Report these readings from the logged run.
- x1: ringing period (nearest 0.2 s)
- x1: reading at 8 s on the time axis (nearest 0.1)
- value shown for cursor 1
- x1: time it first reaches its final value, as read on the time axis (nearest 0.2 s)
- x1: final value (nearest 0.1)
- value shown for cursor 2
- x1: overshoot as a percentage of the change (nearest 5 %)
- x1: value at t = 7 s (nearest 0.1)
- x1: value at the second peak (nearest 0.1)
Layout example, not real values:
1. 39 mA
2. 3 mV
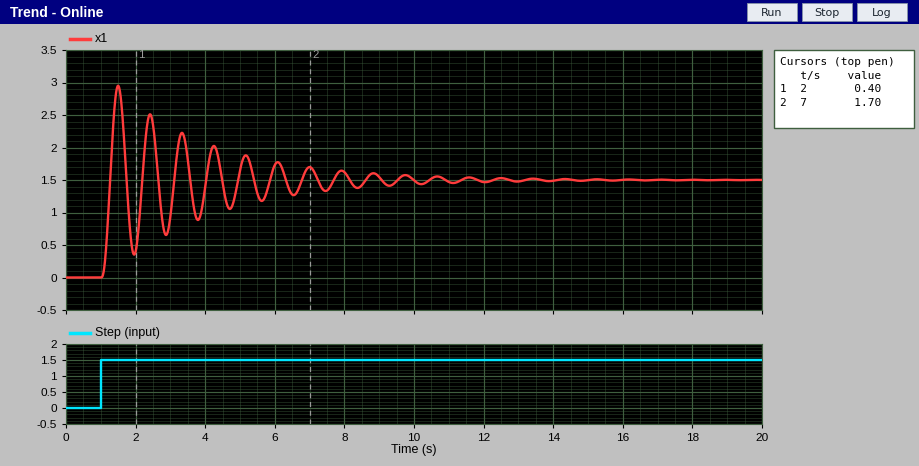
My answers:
1. 1.0 s
2. 1.6
3. 0.40
4. 1.2 s
5. 1.5
6. 1.70
7. 95 %
8. 1.7
9. 2.5
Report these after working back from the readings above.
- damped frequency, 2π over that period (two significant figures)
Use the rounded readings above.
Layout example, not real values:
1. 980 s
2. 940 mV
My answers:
1. 6.3 rad/s
